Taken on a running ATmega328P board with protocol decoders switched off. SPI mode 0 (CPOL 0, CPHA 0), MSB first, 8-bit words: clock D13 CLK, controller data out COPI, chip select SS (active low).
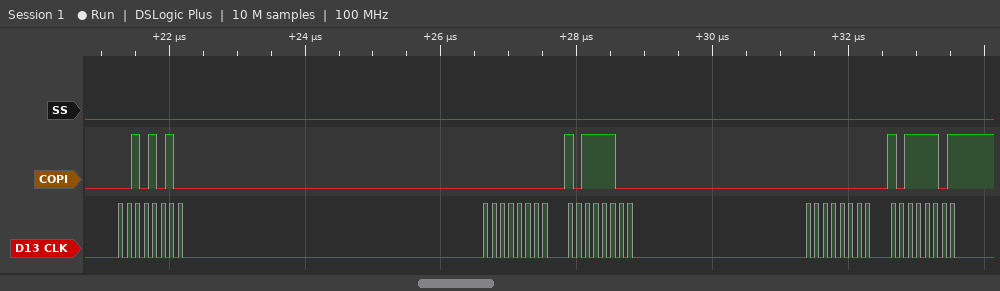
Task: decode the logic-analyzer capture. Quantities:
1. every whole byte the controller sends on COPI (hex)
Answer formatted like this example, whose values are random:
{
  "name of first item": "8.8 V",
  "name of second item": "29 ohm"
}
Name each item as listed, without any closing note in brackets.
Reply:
{
  "every whole byte the controller sends on COPI": "2A 00 BC 00 BD"
}
